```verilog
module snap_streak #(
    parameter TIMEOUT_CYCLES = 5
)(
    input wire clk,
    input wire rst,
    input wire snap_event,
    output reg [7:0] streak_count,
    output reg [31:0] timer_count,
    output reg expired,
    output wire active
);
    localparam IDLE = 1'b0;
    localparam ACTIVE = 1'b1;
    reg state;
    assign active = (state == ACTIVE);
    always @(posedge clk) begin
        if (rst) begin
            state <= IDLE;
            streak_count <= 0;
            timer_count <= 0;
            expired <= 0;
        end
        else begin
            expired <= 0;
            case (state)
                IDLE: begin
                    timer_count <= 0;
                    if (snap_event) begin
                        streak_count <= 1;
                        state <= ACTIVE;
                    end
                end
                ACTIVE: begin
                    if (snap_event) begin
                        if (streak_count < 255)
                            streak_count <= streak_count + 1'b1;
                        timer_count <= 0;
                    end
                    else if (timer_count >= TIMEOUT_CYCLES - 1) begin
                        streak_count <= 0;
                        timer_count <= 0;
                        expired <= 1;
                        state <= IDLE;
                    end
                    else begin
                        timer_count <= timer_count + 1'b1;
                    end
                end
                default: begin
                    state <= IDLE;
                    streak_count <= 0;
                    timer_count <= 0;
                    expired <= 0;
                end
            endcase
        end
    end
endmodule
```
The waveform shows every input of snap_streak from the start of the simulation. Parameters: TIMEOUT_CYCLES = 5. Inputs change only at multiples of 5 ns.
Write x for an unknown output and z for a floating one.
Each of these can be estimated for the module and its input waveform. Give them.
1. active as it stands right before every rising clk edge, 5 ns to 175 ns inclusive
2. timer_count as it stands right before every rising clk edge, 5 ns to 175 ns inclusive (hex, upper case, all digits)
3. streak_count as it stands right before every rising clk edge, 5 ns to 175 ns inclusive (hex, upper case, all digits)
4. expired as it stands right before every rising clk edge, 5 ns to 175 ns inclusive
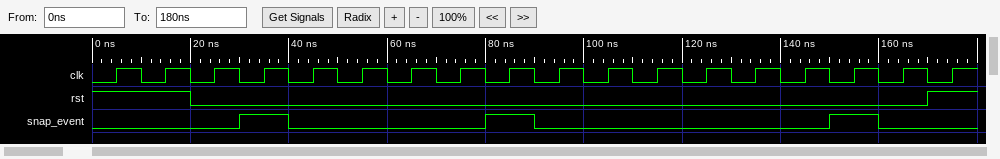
x 0 0 0 1 1 1 1 1 1 1 1 1 1 0 0 1 1
x, 00000000, 00000000, 00000000, 00000000, 00000001, 00000002, 00000003, 00000004, 00000000, 00000001, 00000002, 00000003, 00000004, 00000000, 00000000, 00000000, 00000001
x, 00, 00, 00, 01, 01, 01, 01, 01, 02, 02, 02, 02, 02, 00, 00, 01, 01
x 0 0 0 0 0 0 0 0 0 0 0 0 0 1 0 0 0
